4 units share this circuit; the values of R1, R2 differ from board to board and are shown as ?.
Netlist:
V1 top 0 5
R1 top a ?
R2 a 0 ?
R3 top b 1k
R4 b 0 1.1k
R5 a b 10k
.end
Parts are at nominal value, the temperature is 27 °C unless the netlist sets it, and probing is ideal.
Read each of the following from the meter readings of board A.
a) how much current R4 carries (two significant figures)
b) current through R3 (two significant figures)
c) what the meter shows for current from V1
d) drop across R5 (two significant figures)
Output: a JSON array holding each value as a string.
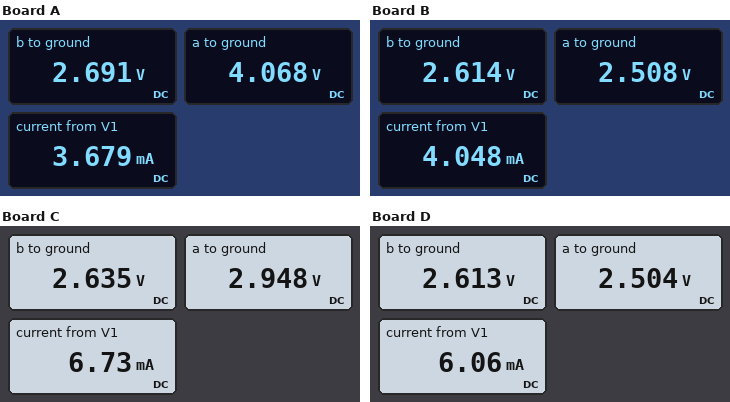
["2.4 mA", "2.3 mA", "3.679 mA", "1.4 V"]
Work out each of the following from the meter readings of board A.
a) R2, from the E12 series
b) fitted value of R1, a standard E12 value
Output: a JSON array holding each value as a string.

["3.3 kΩ", "680 Ω"]
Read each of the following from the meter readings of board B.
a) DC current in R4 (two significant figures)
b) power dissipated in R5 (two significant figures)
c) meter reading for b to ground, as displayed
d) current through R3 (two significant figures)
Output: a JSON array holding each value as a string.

["2.4 mA", "1.1 µW", "2.614 V", "2.4 mA"]
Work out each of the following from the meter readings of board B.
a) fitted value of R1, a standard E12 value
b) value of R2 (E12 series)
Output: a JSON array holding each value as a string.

["1.5 kΩ", "1.5 kΩ"]
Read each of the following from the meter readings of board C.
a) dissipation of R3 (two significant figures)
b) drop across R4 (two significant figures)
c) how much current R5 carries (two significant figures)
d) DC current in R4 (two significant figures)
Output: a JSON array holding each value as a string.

["5.6 mW", "2.6 V", "31 µA", "2.4 mA"]
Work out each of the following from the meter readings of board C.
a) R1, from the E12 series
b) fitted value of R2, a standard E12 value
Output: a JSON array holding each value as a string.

["470 Ω", "680 Ω"]
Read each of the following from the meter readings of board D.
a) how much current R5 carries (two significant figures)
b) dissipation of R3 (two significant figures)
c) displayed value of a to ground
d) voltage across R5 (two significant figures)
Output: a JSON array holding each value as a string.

["11 µA", "5.7 mW", "2.504 V", "110 mV"]
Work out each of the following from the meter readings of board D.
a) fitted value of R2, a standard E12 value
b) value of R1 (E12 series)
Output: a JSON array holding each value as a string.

["680 Ω", "680 Ω"]
